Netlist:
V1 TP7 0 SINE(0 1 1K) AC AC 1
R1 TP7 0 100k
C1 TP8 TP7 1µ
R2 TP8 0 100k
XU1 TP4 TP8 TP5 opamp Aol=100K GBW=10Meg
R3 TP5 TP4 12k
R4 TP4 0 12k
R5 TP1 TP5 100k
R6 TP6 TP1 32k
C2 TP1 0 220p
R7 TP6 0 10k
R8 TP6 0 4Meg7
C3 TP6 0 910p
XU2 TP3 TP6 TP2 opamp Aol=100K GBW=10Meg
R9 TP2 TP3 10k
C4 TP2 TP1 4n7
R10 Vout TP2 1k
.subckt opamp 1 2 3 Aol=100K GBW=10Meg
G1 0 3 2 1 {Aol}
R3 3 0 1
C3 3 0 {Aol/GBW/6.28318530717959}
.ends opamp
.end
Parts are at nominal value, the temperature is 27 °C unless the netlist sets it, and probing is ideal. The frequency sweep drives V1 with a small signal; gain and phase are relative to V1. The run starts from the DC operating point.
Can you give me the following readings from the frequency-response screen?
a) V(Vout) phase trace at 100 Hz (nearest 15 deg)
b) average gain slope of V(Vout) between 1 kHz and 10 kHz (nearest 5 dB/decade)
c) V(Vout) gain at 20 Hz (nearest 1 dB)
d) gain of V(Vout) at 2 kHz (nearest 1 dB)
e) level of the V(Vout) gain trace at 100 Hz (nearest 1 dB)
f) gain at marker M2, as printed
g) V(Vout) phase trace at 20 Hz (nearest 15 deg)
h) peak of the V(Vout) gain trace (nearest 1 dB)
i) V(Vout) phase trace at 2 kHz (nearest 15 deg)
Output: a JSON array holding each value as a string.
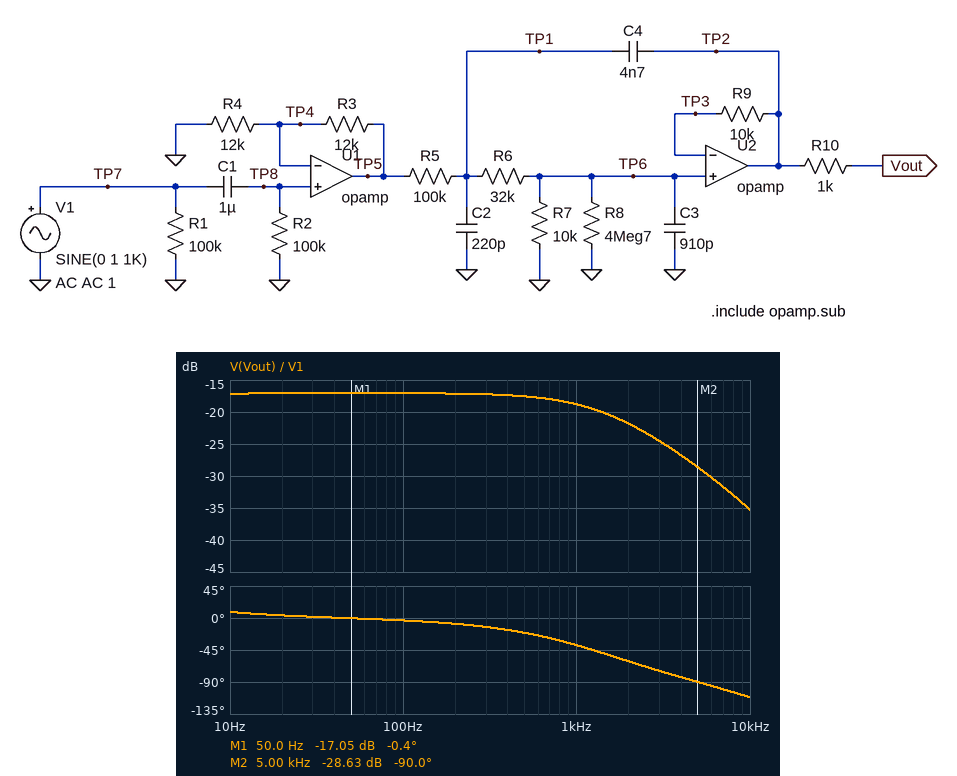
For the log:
["0 deg", "-15 dB/decade", "-17 dB", "-22 dB", "-17 dB", "-28.63 dB", "0 deg", "-17 dB", "-60 deg"]
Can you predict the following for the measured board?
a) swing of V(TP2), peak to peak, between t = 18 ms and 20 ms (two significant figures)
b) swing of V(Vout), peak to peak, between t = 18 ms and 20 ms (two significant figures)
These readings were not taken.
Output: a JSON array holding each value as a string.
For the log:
["230 mV", "230 mV"]
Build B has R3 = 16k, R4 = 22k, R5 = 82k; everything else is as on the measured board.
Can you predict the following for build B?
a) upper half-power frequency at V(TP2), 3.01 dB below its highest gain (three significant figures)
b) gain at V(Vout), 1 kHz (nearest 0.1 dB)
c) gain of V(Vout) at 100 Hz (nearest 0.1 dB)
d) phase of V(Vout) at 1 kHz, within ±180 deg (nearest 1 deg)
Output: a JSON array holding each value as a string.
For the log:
["1.51 kHz", "-18.7 dB", "-17.2 dB", "-37 deg"]
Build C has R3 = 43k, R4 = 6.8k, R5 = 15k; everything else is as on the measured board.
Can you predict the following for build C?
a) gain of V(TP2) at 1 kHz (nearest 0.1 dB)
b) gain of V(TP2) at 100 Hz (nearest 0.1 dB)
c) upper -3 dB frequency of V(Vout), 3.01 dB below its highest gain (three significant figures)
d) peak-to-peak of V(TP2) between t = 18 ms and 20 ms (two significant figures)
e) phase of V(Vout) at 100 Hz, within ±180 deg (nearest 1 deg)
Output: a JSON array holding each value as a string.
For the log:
["1.9 dB", "2.2 dB", "3.78 kHz", "2.5 V", "-1 deg"]
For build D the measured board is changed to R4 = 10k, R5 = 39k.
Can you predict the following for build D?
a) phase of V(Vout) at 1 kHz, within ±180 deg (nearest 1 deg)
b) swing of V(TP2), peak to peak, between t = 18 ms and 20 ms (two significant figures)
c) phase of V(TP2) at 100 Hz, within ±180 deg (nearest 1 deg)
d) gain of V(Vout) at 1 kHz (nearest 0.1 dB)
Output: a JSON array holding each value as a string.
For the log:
["-29 deg", "490 mV", "-2 deg", "-12.2 dB"]
